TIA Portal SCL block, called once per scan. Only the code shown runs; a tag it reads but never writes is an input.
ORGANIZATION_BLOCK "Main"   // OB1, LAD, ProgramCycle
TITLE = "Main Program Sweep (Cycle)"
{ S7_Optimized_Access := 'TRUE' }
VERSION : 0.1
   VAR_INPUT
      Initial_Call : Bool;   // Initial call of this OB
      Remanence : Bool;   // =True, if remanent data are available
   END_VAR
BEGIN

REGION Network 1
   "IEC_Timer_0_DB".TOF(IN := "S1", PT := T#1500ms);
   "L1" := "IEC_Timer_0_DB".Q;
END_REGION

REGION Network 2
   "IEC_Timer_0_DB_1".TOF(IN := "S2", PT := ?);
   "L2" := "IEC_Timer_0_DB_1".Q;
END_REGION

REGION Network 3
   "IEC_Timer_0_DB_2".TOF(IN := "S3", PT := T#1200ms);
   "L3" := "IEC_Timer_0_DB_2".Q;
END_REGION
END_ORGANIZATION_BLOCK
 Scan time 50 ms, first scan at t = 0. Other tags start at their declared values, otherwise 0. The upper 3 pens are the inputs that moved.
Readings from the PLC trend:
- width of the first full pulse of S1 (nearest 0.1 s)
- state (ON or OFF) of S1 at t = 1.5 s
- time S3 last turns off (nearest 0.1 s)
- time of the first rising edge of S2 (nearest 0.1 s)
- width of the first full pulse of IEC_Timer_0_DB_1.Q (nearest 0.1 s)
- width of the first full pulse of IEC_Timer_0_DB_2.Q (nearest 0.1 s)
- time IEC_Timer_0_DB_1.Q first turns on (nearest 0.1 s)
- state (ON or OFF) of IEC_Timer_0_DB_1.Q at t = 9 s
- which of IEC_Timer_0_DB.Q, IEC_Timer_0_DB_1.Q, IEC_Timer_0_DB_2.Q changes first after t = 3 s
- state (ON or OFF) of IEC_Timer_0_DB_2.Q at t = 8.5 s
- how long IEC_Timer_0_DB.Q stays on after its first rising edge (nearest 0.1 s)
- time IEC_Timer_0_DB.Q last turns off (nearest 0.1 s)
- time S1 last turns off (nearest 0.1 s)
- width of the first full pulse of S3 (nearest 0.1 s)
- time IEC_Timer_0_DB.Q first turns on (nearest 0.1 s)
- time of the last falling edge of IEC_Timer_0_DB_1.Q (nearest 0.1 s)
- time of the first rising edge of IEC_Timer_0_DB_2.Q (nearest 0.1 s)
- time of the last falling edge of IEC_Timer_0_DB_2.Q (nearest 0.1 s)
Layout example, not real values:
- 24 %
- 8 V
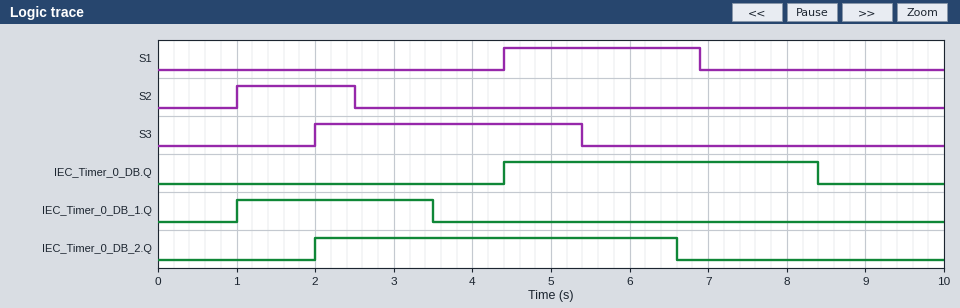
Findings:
- 2.5 s
- OFF
- 5.4 s
- 1.0 s
- 2.5 s
- 4.6 s
- 1.0 s
- OFF
- IEC_Timer_0_DB_1.Q
- OFF
- 4.0 s
- 8.4 s
- 6.9 s
- 3.4 s
- 4.4 s
- 3.5 s
- 2.0 s
- 6.6 s
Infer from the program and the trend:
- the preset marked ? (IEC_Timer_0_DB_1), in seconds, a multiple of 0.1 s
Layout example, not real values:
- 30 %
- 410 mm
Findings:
- 1.0 s
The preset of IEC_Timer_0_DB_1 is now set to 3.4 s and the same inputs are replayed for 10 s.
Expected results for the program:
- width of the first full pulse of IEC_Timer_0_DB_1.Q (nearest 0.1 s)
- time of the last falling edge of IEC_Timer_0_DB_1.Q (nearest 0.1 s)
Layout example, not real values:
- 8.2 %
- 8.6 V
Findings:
- 4.9 s
- 5.9 s
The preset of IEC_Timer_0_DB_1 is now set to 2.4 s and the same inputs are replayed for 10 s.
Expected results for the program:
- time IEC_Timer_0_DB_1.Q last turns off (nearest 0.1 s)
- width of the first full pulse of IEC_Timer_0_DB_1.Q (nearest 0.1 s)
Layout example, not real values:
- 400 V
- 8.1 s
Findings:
- 4.9 s
- 3.9 s
